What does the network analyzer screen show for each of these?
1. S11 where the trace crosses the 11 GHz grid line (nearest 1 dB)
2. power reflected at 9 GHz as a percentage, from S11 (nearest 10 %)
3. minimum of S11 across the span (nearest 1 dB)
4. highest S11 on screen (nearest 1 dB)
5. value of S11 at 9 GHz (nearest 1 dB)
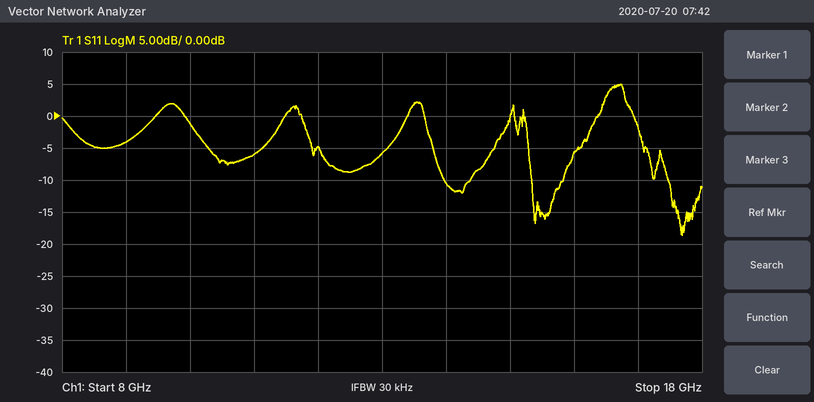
-6 dB
40 %
-19 dB
5 dB
-4 dB
